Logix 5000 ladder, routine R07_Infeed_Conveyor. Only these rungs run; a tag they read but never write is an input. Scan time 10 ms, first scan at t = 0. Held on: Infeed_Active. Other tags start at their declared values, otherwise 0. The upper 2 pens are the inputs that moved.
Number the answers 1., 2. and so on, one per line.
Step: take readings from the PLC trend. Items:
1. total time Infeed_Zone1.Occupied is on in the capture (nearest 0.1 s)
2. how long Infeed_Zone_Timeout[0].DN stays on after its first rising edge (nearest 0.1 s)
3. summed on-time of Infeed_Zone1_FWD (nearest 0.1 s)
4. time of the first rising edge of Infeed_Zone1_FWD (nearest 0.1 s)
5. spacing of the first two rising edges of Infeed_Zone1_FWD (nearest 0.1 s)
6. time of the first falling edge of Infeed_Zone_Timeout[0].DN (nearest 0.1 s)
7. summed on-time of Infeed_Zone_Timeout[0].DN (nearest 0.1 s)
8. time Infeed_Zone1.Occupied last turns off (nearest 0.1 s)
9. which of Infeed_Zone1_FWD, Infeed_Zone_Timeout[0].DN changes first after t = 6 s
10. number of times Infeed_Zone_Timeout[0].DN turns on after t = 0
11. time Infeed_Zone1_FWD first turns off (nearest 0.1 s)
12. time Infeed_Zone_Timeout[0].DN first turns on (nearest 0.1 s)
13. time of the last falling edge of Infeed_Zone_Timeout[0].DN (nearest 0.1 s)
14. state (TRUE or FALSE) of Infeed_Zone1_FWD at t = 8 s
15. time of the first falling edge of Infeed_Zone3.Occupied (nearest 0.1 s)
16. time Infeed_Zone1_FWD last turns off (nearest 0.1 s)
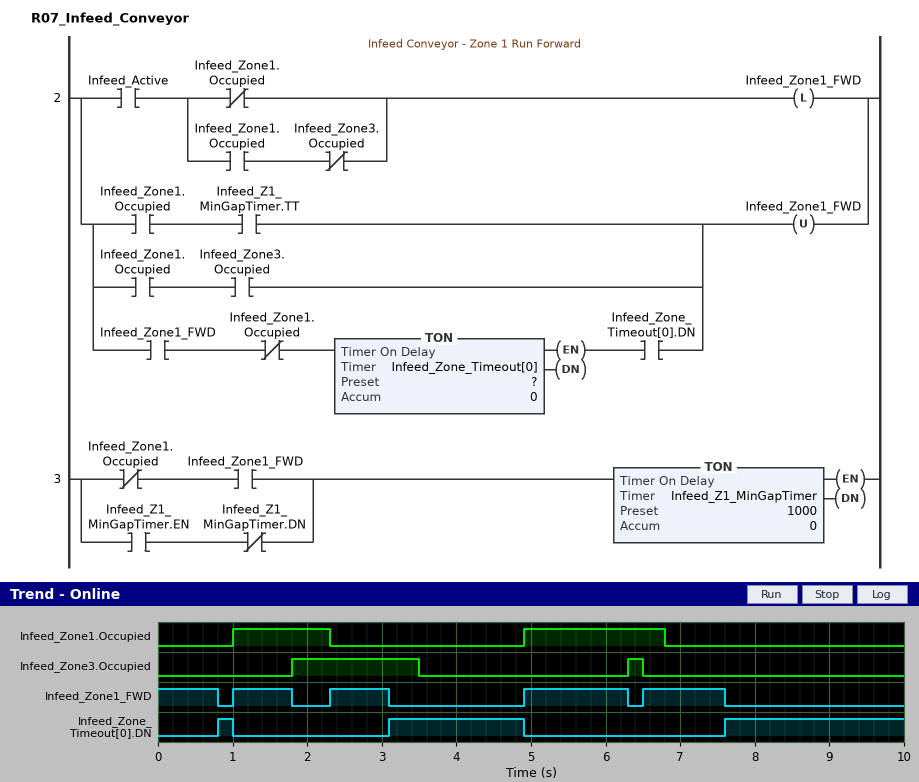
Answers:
1. 3.2 s
2. 0.2 s
3. 4.9 s
4. 1.0 s
5. 1.3 s
6. 1.0 s
7. 4.4 s
8. 6.8 s
9. Infeed_Zone1_FWD
10. 3
11. 0.8 s
12. 0.8 s
13. 4.9 s
14. FALSE
15. 3.5 s
16. 7.6 s
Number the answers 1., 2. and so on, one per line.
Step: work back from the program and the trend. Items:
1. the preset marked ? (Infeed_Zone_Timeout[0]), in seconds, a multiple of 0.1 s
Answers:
1. 0.8 s
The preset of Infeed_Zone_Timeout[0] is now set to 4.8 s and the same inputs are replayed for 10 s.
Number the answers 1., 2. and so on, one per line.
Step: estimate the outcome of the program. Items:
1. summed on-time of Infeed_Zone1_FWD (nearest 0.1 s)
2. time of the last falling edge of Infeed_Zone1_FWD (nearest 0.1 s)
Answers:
1. 9.3 s
2. 6.3 s
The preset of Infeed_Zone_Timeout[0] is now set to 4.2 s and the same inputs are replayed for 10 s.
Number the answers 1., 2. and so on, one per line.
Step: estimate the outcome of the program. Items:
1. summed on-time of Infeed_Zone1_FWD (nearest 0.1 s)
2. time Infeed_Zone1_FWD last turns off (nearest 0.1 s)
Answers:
1. 9.3 s
2. 6.3 s
